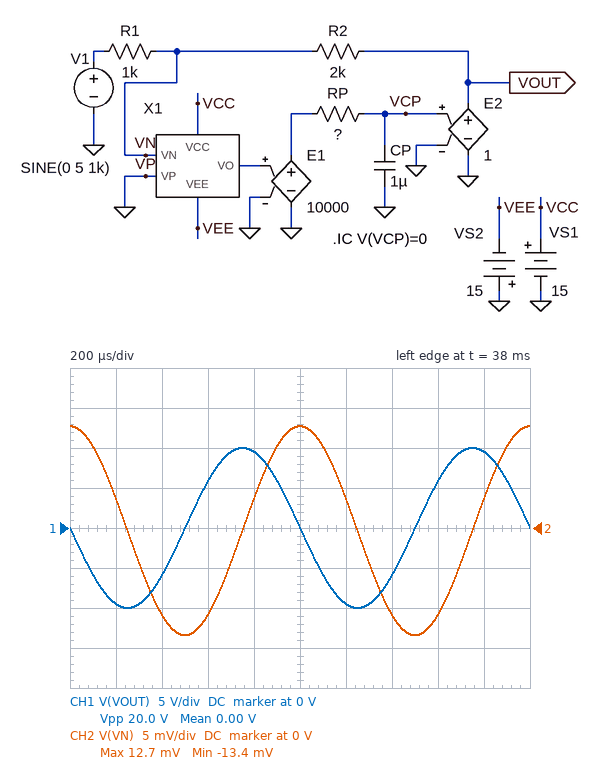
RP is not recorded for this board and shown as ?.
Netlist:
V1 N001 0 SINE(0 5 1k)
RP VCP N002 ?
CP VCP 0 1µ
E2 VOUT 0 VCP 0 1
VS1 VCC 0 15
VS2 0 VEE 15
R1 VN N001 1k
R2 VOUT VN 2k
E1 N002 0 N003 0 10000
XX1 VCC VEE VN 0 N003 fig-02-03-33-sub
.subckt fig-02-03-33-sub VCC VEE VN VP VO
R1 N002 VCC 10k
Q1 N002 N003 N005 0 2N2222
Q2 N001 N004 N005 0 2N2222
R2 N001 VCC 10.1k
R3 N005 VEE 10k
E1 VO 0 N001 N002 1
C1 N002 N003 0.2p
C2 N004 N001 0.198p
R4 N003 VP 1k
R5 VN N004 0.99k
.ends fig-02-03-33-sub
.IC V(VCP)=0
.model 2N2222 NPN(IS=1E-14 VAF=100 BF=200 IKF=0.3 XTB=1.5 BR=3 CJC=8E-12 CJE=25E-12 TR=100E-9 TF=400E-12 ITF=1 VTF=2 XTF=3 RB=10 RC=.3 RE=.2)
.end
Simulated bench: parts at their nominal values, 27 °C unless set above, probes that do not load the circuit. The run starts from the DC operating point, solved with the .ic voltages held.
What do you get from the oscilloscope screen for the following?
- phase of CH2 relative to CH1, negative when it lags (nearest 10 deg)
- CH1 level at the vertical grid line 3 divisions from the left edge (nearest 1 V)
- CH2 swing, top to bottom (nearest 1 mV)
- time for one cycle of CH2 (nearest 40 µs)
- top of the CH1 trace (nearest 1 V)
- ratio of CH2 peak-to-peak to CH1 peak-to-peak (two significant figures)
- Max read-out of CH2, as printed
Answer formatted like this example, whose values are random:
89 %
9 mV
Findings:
-90 deg
6 V
26 mV
1.00 ms
10 V
0.0013
12.7 mV
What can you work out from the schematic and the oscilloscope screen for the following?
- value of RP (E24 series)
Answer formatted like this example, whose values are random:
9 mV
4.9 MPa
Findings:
470 kΩ
